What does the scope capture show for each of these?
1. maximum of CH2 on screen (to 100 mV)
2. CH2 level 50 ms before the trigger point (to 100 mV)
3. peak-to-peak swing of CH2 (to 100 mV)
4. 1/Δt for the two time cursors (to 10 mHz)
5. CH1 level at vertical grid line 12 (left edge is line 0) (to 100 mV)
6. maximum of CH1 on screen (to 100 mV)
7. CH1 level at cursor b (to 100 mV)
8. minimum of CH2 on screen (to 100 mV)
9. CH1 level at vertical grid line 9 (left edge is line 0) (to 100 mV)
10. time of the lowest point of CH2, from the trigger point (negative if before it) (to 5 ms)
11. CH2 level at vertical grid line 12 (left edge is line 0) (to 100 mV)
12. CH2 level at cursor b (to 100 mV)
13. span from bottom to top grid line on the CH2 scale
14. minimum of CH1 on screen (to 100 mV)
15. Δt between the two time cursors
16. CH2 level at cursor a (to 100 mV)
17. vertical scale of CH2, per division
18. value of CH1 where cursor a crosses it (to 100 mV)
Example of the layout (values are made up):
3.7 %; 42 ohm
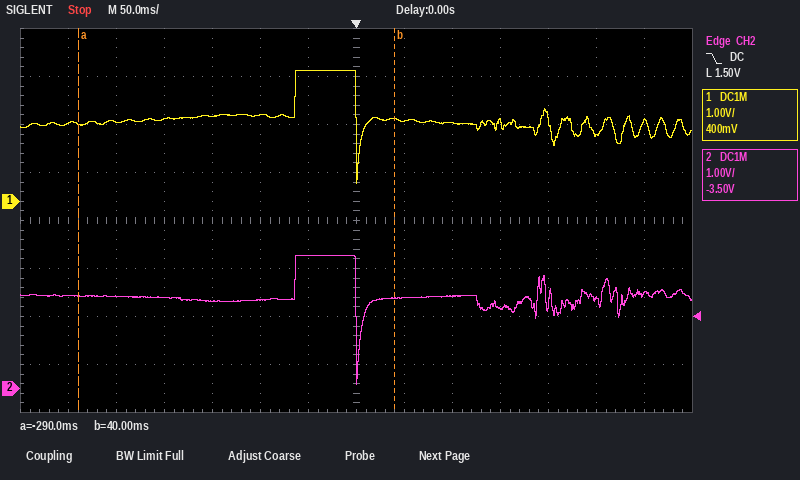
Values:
2.8 V; 2.8 V; 2.7 V; 3.03 Hz; 1.4 V; 2.7 V; 1.7 V; 100 mV; 1.6 V; 0 ms; 1.9 V; 1.9 V; 8 V; 400 mV; 330 ms; 1.9 V; 1 V; 1.6 V
